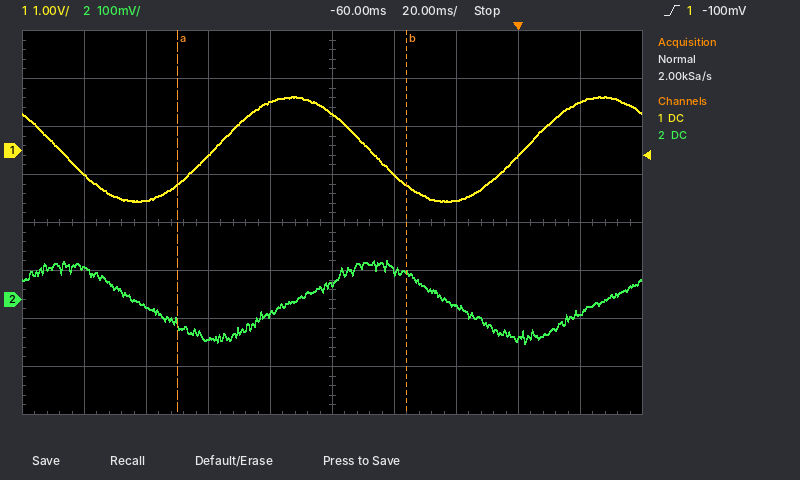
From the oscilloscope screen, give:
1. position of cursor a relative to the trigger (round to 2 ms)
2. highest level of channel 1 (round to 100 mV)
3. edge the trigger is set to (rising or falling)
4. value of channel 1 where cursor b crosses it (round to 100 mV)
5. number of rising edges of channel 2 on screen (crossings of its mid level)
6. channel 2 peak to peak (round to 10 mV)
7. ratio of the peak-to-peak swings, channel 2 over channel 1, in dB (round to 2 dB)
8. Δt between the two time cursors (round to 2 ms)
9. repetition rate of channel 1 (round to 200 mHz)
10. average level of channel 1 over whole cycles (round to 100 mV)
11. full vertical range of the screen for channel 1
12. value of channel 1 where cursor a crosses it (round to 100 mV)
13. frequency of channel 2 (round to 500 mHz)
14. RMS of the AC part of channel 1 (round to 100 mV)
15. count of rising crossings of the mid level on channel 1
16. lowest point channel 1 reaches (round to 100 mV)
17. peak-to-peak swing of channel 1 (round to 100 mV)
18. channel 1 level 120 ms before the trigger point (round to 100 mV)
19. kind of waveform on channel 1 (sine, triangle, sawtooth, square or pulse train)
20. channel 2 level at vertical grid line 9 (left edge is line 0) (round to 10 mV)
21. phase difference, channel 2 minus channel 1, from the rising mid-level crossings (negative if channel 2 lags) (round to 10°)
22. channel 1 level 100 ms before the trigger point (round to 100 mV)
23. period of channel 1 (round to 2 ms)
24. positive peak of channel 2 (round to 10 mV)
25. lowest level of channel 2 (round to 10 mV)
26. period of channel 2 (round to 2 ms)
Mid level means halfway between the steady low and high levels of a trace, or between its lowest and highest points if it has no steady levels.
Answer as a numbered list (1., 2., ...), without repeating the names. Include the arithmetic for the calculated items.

1. -110 ms
2. 1.1 V
3. rising
4. -700 mV
5. 2
6. 80 mV − (-90 mV) = 170 mV
7. 20 log10(170 mV / 2.2 V) ≈ -22 dB
8. 74 ms
9. 1 / 100 ms ≈ 10.0 Hz
10. (1.1 V + (-1.1 V)) / 2 ≈ 0.0 V
11. 8 V
12. -700 mV
13. 1 / 100 ms ≈ 10.0 Hz
14. 2.2 V / (2√2) ≈ 778 mV, so 800 mV to the nearest 100 mV
15. 2
16. -1.1 V
17. 1.1 V − (-1.1 V) = 2.2 V
18. -1.0 V
19. sine
20. -30 mV
21. -90°
22. -100 mV
23. 100 ms
24. 80 mV
25. -90 mV
26. 100 ms
